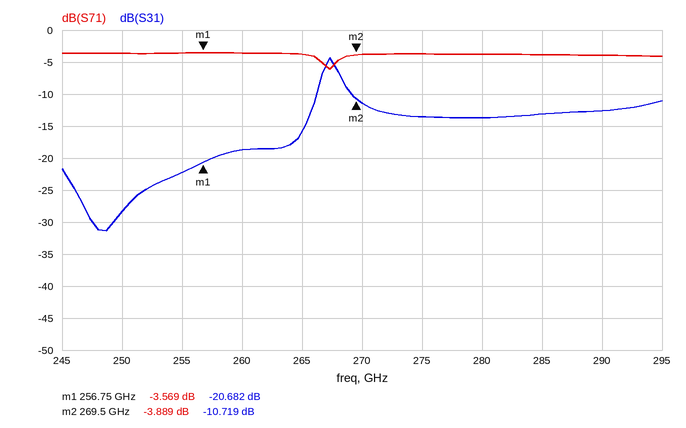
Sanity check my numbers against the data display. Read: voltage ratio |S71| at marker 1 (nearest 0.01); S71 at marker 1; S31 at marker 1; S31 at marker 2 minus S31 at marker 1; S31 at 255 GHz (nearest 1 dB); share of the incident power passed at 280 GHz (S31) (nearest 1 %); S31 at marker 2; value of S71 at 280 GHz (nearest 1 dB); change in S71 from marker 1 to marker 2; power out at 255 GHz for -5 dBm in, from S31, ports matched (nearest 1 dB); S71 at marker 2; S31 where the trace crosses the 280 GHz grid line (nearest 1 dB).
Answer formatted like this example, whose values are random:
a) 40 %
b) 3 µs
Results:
a) 0.66
b) -3.569 dB
c) -20.682 dB
d) 9.963 dB
e) -22 dB
f) 4 %
g) -10.719 dB
h) -4 dB
i) -0.320 dB
j) -27 dBm
k) -3.889 dB
l) -14 dB
